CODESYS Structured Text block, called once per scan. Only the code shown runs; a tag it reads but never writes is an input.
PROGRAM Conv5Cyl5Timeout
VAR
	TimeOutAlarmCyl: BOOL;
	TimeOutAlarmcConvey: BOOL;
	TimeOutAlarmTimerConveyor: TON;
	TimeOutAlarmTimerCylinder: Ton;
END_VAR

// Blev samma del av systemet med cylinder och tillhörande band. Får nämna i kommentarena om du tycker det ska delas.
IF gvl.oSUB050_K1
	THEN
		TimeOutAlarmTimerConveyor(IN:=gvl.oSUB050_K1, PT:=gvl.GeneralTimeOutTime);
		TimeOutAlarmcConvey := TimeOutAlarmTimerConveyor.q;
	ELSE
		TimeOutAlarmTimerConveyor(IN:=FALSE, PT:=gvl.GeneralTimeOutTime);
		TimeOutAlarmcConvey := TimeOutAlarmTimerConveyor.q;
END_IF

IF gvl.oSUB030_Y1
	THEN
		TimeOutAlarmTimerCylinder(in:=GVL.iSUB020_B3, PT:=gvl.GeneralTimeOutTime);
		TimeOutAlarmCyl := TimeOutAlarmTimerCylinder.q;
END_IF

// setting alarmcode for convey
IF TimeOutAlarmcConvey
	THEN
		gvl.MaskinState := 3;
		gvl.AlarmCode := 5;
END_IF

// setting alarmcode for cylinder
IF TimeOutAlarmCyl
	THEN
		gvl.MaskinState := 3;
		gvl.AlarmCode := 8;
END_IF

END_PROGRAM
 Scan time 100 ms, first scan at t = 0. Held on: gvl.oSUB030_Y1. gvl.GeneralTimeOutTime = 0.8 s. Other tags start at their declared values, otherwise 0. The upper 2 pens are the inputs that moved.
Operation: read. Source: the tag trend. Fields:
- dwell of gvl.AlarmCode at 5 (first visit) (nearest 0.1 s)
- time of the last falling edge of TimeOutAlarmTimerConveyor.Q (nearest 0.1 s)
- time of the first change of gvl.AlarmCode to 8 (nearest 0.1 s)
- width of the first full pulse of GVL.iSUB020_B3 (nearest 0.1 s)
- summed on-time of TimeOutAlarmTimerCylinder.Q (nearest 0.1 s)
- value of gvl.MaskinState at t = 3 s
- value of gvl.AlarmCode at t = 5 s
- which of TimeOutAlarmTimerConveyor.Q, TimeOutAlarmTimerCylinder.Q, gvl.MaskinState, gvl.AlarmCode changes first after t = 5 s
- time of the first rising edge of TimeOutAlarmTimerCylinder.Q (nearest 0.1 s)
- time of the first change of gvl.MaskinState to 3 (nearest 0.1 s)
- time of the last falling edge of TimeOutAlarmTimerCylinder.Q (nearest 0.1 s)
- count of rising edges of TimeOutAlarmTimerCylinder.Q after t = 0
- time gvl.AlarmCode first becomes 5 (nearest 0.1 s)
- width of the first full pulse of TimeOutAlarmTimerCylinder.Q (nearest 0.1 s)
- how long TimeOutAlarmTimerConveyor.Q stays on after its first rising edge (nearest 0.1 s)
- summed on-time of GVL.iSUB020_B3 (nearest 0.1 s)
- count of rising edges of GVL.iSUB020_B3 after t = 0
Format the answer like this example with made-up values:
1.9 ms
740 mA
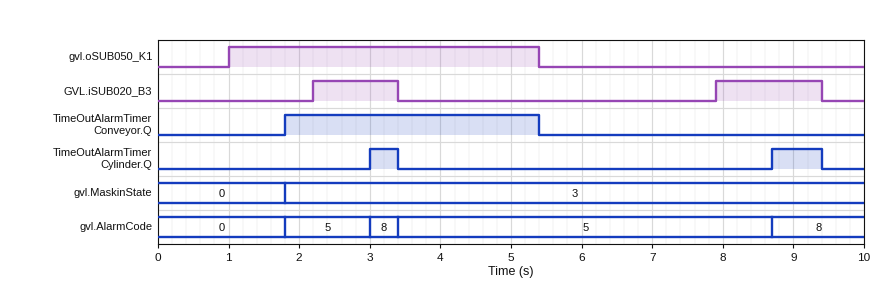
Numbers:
1.2 s
5.4 s
3.0 s
1.2 s
1.1 s
3
5
TimeOutAlarmTimerConveyor.Q
3.0 s
1.8 s
9.4 s
2
1.8 s
0.4 s
3.6 s
2.7 s
2
